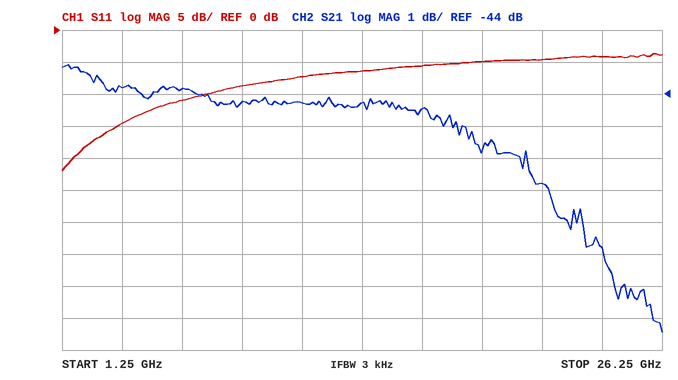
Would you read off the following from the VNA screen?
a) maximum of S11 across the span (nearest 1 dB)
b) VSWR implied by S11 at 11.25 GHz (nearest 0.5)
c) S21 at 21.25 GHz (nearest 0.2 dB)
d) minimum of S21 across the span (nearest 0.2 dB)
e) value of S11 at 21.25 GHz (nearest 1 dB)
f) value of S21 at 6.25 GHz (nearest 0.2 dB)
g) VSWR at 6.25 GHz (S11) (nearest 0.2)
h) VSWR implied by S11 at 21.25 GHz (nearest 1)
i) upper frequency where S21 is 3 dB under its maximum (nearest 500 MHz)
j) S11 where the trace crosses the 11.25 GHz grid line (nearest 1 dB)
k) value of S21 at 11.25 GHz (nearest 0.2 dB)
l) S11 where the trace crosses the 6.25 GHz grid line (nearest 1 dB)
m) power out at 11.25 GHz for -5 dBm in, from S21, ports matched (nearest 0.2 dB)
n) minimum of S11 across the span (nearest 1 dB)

-4 dB
2.5
-46.8 dB
-51.4 dB
-5 dB
-43.8 dB
1.8
4
20.5 GHz
-7 dB
-44.2 dB
-11 dB
-49.2 dBm
-22 dB
